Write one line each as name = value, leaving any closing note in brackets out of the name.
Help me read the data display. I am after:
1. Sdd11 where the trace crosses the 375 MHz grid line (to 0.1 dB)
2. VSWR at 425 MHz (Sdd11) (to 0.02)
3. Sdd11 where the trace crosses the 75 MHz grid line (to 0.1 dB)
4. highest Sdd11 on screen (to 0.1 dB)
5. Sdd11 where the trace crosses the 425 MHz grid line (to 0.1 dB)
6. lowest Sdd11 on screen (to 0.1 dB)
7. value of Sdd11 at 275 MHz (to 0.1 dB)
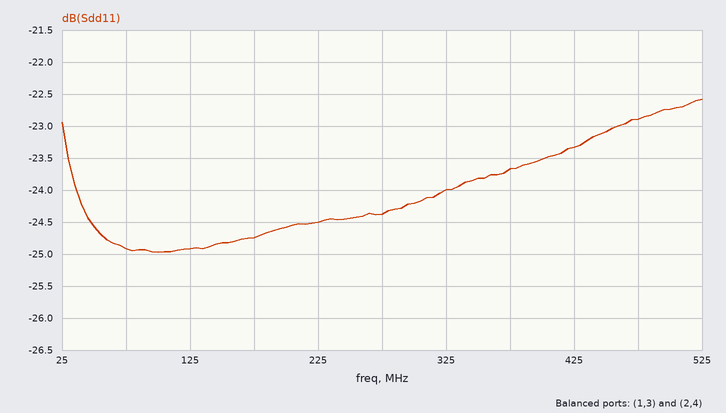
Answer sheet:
Sdd11 where the trace crosses the 375 MHz grid line = -23.7 dB
VSWR at 425 MHz (Sdd11) = 1.14
Sdd11 where the trace crosses the 75 MHz grid line = -24.9 dB
highest Sdd11 on screen = -22.6 dB
Sdd11 where the trace crosses the 425 MHz grid line = -23.3 dB
lowest Sdd11 on screen = -25.0 dB
value of Sdd11 at 275 MHz = -24.4 dB
